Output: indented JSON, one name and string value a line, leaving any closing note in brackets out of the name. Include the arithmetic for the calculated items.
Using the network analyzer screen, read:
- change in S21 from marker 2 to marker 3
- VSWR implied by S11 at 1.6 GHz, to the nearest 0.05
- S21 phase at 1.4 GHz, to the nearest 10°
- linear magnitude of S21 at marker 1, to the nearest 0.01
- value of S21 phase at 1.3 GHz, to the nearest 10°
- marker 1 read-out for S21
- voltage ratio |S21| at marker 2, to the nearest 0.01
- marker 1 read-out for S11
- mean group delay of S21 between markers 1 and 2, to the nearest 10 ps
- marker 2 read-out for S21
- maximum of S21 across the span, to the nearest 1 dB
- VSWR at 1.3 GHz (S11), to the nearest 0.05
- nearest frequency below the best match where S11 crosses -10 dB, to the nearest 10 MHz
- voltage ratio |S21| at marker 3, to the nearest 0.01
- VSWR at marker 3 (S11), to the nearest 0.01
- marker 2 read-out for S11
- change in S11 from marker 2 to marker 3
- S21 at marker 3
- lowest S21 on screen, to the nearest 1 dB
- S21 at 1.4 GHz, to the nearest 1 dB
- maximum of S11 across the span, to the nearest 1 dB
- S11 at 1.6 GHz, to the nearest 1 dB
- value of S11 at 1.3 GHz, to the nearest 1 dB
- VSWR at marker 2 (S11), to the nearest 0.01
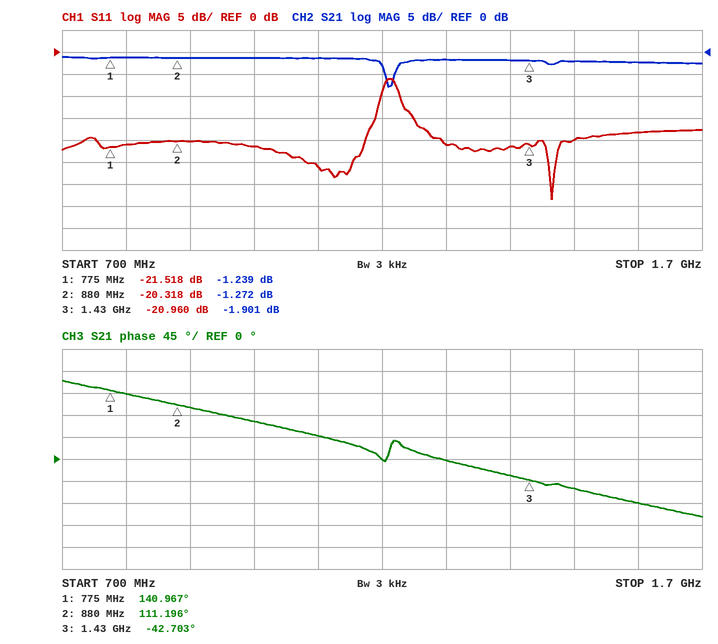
{
  "change in S21 from marker 2 to marker 3": "-1.901 − (-1.272) = -0.629 dB",
  "VSWR implied by S11 at 1.6 GHz, to the nearest 0.05": "|Γ| = 10^(-18/20) = 0.1259; VSWR = (1 + 0.1259)/(1 − 0.1259) ≈ 1.29, so 1.30 to the nearest 0.05",
  "S21 phase at 1.4 GHz, to the nearest 10°": "-30°",
  "linear magnitude of S21 at marker 1, to the nearest 0.01": "10^(-1.239/20) ≈ 0.87",
  "value of S21 phase at 1.3 GHz, to the nearest 10°": "0°",
  "marker 1 read-out for S21": "-1.239 dB",
  "voltage ratio |S21| at marker 2, to the nearest 0.01": "10^(-1.272/20) ≈ 0.86",
  "marker 1 read-out for S11": "-21.518 dB",
  "mean group delay of S21 between markers 1 and 2, to the nearest 10 ps": "−(111.196° − (140.967°))/(360° × 105 MHz) ≈ 788 ps, so 790 ps to the nearest 10 ps",
  "marker 2 read-out for S21": "-1.272 dB",
  "maximum of S21 across the span, to the nearest 1 dB": "-1 dB",
  "VSWR at 1.3 GHz (S11), to the nearest 0.05": "|Γ| = 10^(-21/20) = 0.0891; VSWR = (1 + 0.0891)/(1 − 0.0891) ≈ 1.20",
  "nearest frequency below the best match where S11 crosses -10 dB, to the nearest 10 MHz": "1.23 GHz",
  "voltage ratio |S21| at marker 3, to the nearest 0.01": "10^(-1.901/20) ≈ 0.80",
  "VSWR at marker 3 (S11), to the nearest 0.01": "(1 + 0.0895)/(1 − 0.0895) ≈ 1.20",
  "marker 2 read-out for S11": "-20.318 dB",
  "change in S11 from marker 2 to marker 3": "-20.96 − (-20.318) = -0.642 dB",
  "S21 at marker 3": "-1.901 dB",
  "lowest S21 on screen, to the nearest 1 dB": "-8 dB",
  "S21 at 1.4 GHz, to the nearest 1 dB": "-2 dB",
  "maximum of S11 across the span, to the nearest 1 dB": "-6 dB",
  "S11 at 1.6 GHz, to the nearest 1 dB": "-18 dB",
  "value of S11 at 1.3 GHz, to the nearest 1 dB": "-21 dB",
  "VSWR at marker 2 (S11), to the nearest 0.01": "(1 + 0.0964)/(1 − 0.0964) ≈ 1.21"
}
